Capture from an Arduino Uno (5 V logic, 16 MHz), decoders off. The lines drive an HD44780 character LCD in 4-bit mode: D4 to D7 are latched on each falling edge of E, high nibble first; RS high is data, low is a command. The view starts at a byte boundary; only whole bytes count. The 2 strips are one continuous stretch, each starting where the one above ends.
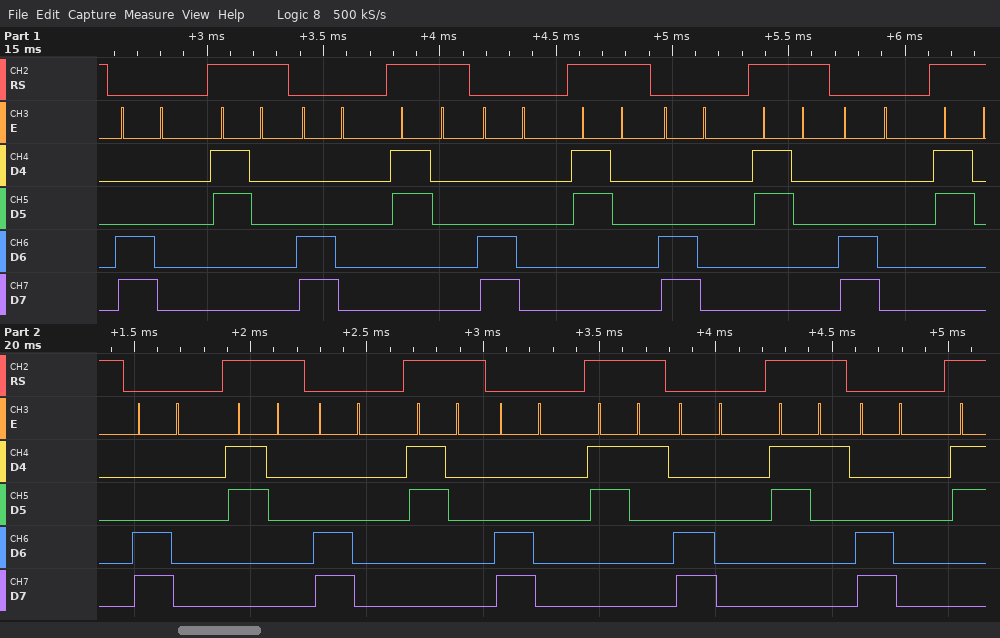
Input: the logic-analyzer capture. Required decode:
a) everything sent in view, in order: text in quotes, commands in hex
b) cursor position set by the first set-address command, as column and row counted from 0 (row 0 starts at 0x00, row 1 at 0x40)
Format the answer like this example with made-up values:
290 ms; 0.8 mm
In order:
0xC0 "0" 0xC0 "0" 0xC0 "0" 0xC0 "0" 0xC0 "0" 0xC0 "0" 0xC0 "0" 0xC0 "1" 0xC0 "1" 0xC0; column 0, row 1
